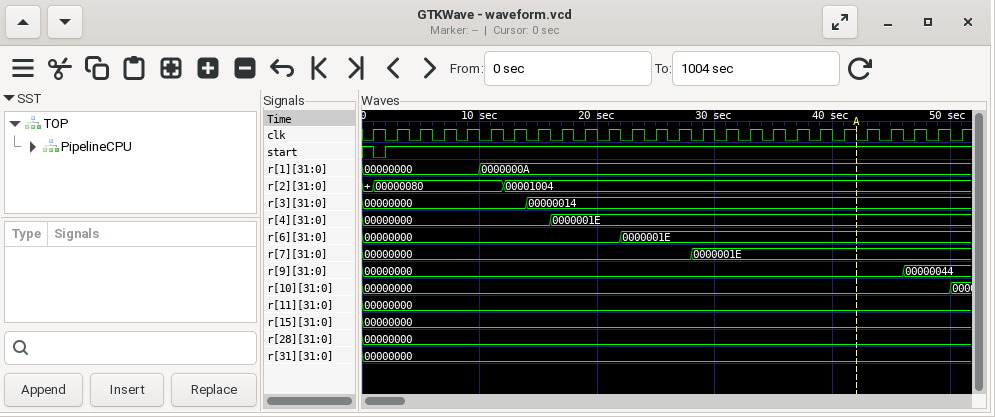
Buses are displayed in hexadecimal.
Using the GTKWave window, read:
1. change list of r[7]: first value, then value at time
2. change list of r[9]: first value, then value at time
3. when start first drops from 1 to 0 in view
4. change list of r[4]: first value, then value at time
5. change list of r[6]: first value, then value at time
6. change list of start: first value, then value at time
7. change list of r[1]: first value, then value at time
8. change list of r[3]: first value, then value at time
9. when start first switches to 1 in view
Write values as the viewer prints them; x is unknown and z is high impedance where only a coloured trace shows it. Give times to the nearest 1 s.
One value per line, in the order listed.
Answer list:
00000000, 0000001E at 28 s
00000000, 00000044 at 46 s
1 s
00000000, 0000001E at 16 s
00000000, 0000001E at 22 s
1, 0 at 1 s, 1 at 2 s
00000000, 0000000A at 10 s
00000000, 00000014 at 14 s
2 s
